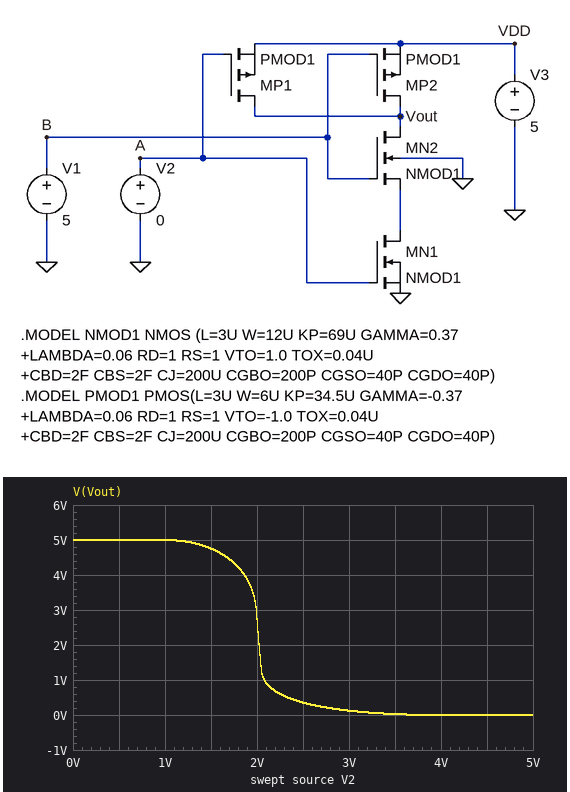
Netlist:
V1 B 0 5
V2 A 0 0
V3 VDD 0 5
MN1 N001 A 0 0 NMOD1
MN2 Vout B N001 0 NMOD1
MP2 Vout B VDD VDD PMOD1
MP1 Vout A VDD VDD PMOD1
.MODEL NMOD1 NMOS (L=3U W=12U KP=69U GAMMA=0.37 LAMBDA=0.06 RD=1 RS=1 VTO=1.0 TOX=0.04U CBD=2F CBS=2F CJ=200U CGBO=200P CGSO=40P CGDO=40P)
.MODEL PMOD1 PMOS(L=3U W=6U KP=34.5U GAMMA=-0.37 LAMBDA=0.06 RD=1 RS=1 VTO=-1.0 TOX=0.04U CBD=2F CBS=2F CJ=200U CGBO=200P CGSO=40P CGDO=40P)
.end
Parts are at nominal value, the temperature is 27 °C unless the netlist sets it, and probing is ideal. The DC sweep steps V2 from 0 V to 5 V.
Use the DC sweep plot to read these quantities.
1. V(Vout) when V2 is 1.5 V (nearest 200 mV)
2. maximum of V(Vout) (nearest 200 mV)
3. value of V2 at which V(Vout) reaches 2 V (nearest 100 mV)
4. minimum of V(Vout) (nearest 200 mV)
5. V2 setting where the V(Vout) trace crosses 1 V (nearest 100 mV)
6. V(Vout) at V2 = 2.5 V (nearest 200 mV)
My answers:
4.8 V
5.0 V
2.0 V
0 V
2.1 V
400 mV
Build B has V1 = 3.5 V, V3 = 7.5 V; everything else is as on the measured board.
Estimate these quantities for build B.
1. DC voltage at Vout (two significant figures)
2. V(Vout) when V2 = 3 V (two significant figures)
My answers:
7.5 V
6.5 V
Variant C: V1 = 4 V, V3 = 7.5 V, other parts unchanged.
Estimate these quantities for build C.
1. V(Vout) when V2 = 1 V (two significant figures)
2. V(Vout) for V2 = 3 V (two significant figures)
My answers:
7.5 V
6.1 V
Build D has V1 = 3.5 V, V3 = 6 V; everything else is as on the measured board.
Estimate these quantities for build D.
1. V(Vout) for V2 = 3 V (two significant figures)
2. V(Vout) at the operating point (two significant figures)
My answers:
1.2 V
6.0 V
